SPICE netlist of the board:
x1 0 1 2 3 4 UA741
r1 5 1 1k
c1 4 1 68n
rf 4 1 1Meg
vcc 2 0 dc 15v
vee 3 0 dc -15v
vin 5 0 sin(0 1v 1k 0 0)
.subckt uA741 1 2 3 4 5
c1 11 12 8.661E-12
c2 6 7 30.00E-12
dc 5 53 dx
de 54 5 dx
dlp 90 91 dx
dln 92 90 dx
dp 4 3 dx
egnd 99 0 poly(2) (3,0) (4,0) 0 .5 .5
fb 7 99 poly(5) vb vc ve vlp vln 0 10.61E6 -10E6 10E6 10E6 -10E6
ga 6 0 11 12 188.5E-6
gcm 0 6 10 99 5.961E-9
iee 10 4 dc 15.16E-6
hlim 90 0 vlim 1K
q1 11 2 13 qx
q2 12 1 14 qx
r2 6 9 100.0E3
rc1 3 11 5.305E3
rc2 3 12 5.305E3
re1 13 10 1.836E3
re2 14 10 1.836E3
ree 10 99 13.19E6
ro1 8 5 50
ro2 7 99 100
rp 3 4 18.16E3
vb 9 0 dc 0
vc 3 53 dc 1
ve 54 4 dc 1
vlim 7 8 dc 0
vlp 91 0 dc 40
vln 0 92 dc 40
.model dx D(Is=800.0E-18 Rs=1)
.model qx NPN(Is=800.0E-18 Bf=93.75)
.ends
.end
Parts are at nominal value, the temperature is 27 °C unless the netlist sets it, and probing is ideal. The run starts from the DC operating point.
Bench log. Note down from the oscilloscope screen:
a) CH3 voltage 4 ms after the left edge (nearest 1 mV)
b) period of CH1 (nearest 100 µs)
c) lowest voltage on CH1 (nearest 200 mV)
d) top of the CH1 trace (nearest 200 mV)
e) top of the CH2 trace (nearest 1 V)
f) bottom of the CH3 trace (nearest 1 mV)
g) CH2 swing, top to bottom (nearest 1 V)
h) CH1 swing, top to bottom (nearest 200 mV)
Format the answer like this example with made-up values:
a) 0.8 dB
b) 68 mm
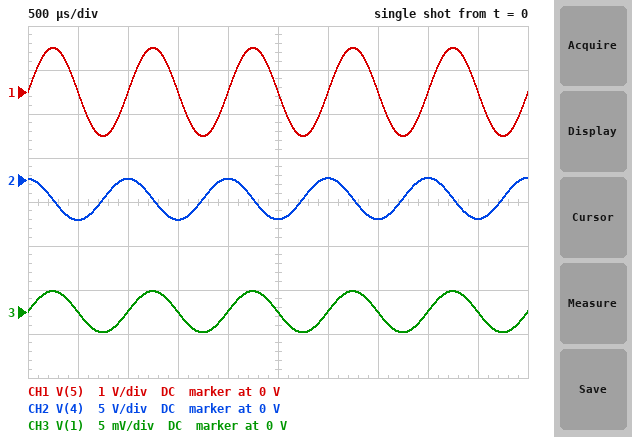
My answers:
a) 0 V
b) 1.0 ms
c) -1.0 V
d) 1.0 V
e) 0 V
f) -2 mV
g) 5 V
h) 2.0 V
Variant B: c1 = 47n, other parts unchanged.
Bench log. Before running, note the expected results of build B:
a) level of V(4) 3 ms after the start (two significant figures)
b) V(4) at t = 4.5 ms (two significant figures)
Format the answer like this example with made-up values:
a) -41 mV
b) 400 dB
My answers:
a) 310 mV
b) -6.3 V
